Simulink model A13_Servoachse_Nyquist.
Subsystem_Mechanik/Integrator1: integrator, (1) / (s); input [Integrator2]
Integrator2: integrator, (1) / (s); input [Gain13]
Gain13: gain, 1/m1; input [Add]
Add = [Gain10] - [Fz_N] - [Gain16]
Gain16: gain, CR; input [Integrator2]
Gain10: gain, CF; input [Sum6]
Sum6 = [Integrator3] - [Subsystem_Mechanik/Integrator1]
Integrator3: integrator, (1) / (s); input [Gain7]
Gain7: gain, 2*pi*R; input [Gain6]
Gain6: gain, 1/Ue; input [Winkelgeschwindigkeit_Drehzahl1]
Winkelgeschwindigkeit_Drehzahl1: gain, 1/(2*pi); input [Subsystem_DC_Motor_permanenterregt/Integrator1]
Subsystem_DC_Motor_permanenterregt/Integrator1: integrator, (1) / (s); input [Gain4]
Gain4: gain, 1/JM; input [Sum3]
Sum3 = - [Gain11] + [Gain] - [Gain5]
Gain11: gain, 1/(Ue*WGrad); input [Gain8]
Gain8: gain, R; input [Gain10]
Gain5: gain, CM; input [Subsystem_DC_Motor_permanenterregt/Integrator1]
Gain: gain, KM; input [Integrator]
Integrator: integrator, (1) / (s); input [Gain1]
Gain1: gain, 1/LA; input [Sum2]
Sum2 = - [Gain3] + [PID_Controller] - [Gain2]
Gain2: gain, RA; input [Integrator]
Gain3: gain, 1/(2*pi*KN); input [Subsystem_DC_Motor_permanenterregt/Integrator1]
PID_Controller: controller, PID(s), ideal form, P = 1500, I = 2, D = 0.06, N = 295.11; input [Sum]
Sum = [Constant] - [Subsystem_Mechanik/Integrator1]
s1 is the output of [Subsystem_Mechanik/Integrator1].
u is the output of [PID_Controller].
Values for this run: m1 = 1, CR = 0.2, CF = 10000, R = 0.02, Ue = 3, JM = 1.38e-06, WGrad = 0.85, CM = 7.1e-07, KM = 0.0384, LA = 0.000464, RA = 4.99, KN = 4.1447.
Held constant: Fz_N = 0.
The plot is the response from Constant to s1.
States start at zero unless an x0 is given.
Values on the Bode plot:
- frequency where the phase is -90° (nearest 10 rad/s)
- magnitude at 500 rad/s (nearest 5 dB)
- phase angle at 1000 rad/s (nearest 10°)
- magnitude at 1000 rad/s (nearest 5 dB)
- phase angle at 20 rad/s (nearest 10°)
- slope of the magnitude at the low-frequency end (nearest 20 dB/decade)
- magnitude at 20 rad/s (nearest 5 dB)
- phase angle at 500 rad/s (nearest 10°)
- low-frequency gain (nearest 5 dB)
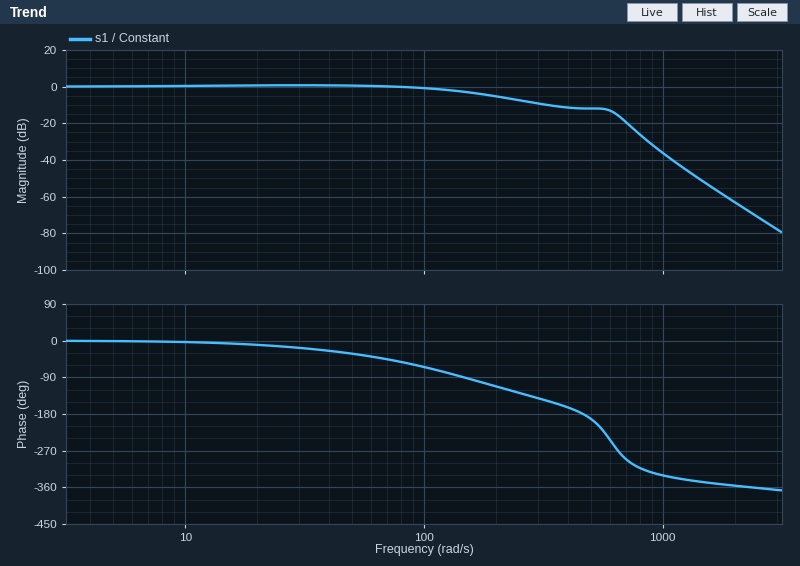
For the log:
150 rad/s
-10 dB
-330°
-35 dB
-10°
0 dB/decade
0 dB
-190°
0 dB
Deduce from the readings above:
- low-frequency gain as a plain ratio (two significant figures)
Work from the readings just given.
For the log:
1.0
